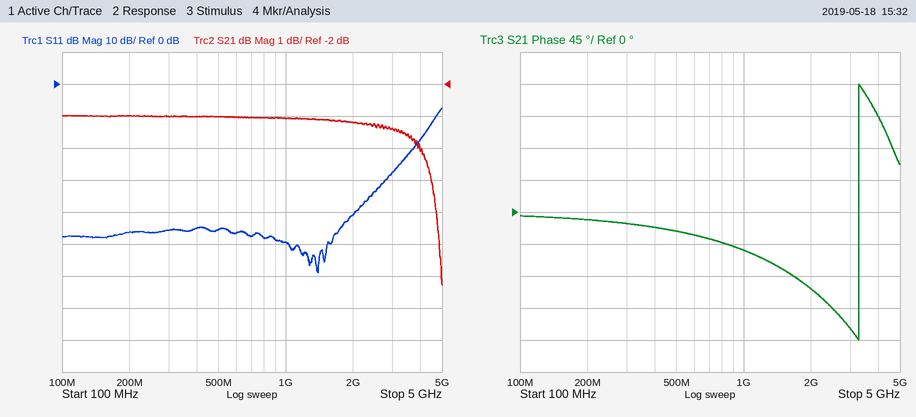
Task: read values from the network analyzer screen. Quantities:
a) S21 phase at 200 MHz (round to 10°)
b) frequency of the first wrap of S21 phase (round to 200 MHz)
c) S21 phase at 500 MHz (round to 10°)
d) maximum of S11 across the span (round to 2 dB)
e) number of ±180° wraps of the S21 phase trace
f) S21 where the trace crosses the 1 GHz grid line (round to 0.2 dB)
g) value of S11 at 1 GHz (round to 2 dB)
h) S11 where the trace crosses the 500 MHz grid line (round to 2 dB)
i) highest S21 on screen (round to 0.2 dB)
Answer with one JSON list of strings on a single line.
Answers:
["-10°", "3.2 GHz", "-30°", "-8 dB", "1", "-3.0 dB", "-50 dB", "-46 dB", "-3.0 dB"]
